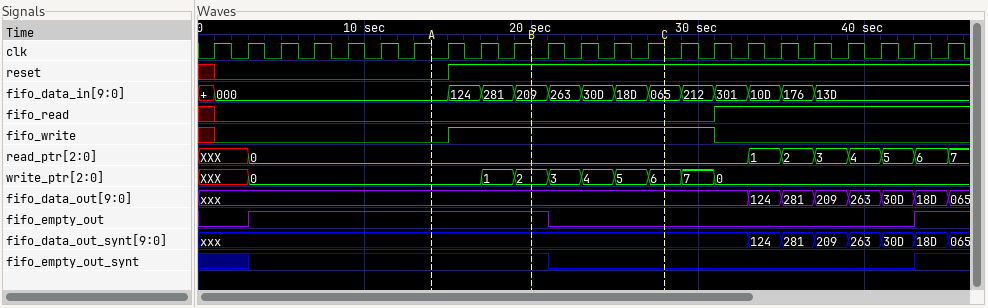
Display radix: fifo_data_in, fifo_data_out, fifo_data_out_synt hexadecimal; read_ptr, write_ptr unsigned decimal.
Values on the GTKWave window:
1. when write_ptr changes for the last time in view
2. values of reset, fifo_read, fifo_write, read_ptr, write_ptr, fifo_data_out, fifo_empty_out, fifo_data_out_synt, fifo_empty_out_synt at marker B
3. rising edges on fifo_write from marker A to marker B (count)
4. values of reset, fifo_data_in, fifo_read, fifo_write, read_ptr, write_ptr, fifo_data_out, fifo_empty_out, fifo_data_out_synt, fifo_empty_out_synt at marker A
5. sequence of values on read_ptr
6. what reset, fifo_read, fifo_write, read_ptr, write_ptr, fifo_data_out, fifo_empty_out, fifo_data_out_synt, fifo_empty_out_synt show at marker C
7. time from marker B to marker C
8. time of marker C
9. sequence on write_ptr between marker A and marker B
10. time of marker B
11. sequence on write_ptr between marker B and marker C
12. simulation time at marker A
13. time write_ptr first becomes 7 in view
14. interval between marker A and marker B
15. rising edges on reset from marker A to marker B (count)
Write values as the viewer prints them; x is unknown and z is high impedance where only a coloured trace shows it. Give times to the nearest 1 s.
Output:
31 s
reset=1, fifo_read=0, fifo_write=1, read_ptr=0, write_ptr=2, fifo_data_out=xxx, fifo_empty_out=1, fifo_data_out_synt=xxx, fifo_empty_out_synt=1
1
reset=0, fifo_data_in=000, fifo_read=0, fifo_write=0, read_ptr=0, write_ptr=0, fifo_data_out=xxx, fifo_empty_out=1, fifo_data_out_synt=xxx, fifo_empty_out_synt=1
XXX, 0, 1, 2, 3, 4, 5, 6, 7
reset=1, fifo_read=0, fifo_write=1, read_ptr=0, write_ptr=6, fifo_data_out=xxx, fifo_empty_out=0, fifo_data_out_synt=xxx, fifo_empty_out_synt=0
8 s
28 s
0, 1, 2
20 s
2, 3, 4, 5, 6
14 s
29 s
6 s
1
